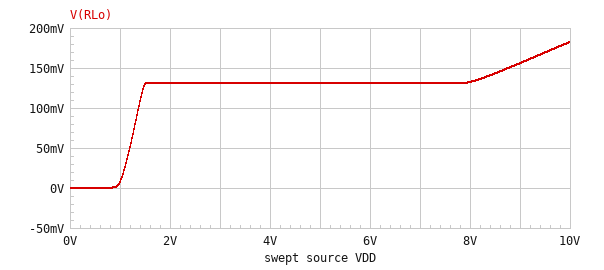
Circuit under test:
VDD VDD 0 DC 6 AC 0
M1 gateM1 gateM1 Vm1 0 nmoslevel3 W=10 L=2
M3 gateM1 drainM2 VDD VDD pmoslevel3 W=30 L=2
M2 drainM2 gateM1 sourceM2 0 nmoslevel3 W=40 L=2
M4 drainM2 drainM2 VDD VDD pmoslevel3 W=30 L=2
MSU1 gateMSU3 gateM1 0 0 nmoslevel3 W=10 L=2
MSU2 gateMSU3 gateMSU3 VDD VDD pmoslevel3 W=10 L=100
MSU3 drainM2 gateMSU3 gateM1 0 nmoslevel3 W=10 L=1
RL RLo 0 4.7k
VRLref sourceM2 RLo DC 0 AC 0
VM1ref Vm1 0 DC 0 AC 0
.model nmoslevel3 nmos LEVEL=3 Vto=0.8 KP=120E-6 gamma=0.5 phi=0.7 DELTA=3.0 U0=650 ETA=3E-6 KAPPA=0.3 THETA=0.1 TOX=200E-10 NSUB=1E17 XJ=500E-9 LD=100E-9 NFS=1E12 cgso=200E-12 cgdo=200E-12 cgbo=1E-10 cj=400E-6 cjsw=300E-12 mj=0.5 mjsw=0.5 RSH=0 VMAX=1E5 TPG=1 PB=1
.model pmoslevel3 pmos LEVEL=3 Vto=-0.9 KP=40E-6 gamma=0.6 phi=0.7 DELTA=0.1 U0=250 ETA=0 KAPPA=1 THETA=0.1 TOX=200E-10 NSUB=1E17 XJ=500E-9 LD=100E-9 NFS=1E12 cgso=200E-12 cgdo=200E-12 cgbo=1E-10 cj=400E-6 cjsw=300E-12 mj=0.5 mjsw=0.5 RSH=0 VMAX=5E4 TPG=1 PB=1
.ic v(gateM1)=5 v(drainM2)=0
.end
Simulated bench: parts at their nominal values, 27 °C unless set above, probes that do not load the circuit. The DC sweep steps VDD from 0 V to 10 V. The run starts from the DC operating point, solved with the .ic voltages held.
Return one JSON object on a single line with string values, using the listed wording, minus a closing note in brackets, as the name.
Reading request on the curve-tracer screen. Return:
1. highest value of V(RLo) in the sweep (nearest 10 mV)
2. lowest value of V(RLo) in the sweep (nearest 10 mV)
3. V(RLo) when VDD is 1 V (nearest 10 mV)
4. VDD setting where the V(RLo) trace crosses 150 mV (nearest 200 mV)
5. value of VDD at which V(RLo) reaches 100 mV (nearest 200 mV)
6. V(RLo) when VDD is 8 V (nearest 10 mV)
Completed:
{"highest value of V(RLo) in the sweep": "180 mV", "lowest value of V(RLo) in the sweep": "0 V", "V(RLo) when VDD is 1 V": "10 mV", "VDD setting where the V(RLo) trace crosses 150 mV": "8.8 V", "value of VDD at which V(RLo) reaches 100 mV": "1.4 V", "V(RLo) when VDD is 8 V": "130 mV"}
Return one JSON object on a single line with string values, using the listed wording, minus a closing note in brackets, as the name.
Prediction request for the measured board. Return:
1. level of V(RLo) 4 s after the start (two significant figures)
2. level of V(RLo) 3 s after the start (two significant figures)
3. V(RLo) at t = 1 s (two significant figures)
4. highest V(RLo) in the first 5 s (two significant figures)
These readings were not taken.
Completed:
{"level of V(RLo) 4 s after the start": "33 mV", "level of V(RLo) 3 s after the start": "23 mV", "V(RLo) at t = 1 s": "6.4 mV", "highest V(RLo) in the first 5 s": "44 mV"}
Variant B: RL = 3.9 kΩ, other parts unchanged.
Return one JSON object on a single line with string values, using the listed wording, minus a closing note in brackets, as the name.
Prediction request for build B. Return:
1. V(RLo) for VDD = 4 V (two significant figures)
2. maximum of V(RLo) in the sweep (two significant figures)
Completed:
{"V(RLo) for VDD = 4 V": "160 mV", "maximum of V(RLo) in the sweep": "170 mV"}
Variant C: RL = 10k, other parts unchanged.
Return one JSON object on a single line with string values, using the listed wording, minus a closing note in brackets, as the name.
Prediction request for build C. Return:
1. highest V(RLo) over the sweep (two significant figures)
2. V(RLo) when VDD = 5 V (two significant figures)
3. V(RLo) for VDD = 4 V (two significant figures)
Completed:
{"highest V(RLo) over the sweep": "220 mV", "V(RLo) when VDD = 5 V": "64 mV", "V(RLo) for VDD = 4 V": "59 mV"}
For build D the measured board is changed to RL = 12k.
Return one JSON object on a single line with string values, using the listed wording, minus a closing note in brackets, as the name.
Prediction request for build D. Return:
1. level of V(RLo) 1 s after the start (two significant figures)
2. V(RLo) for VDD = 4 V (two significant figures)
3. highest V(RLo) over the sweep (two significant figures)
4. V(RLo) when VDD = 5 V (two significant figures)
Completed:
{"level of V(RLo) 1 s after the start": "6.4 mV", "V(RLo) for VDD = 4 V": "49 mV", "highest V(RLo) over the sweep": "230 mV", "V(RLo) when VDD = 5 V": "66 mV"}
